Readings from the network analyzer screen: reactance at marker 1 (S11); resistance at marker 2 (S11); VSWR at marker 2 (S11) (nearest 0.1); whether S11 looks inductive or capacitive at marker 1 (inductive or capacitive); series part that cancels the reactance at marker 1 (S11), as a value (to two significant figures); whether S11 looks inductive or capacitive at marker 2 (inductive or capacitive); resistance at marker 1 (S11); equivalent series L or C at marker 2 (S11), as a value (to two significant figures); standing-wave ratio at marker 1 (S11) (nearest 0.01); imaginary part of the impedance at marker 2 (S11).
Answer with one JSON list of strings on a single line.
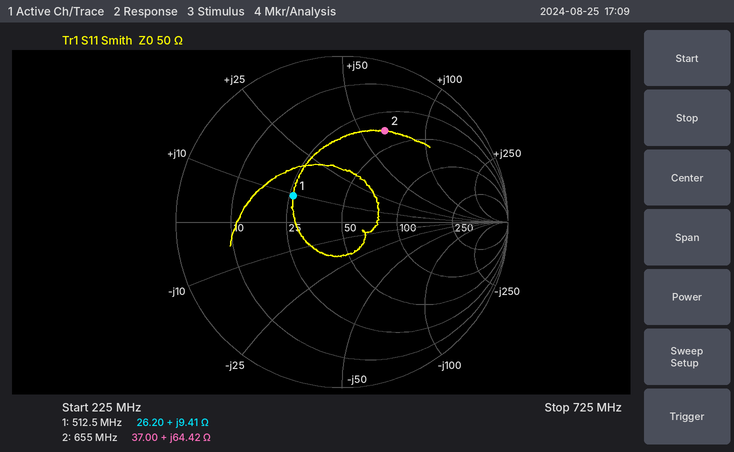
["+9.41 Ω", "37.00 Ω", "4.1", "inductive", "33 pF", "inductive", "26.20 Ω", "16 nH", "2.00", "+64.42 Ω"]
